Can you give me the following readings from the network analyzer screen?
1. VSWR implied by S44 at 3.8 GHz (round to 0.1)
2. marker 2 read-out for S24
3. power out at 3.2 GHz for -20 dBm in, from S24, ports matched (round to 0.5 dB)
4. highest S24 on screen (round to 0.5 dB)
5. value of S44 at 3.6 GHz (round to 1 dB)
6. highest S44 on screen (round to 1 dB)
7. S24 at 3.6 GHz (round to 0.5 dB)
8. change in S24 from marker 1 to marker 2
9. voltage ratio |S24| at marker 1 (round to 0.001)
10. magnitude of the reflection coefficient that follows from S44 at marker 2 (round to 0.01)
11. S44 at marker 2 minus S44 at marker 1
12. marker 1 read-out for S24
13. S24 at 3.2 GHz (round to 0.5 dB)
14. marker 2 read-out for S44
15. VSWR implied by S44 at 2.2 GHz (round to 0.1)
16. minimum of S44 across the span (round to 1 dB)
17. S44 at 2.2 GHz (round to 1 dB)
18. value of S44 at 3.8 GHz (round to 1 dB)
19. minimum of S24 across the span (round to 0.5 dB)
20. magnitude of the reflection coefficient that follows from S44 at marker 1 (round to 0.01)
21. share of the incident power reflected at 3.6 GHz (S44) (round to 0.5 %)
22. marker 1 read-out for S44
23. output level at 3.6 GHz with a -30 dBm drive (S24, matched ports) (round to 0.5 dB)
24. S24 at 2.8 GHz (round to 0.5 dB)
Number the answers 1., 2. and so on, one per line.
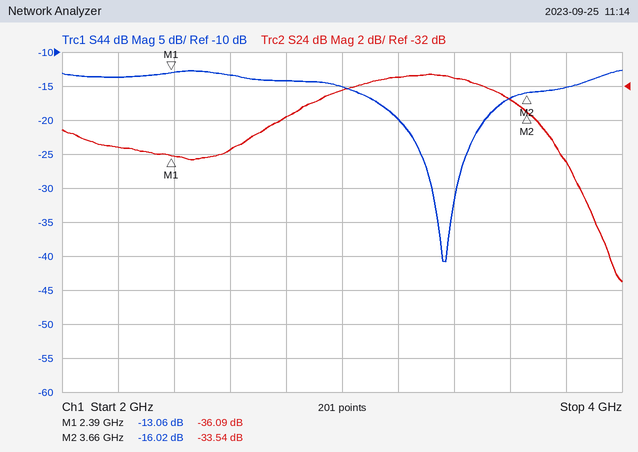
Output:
1. 1.4
2. -33.54 dB
3. -51.5 dBm
4. -31.5 dB
5. -17 dB
6. -13 dB
7. -33.0 dB
8. 2.55 dB
9. 0.016
10. 0.16
11. -2.96 dB
12. -36.09 dB
13. -31.5 dB
14. -16.02 dB
15. 1.5
16. -41 dB
17. -14 dB
18. -15 dB
19. -43.5 dB
20. 0.22
21. 2.0 %
22. -13.06 dB
23. -63.0 dBm
24. -34.0 dB
